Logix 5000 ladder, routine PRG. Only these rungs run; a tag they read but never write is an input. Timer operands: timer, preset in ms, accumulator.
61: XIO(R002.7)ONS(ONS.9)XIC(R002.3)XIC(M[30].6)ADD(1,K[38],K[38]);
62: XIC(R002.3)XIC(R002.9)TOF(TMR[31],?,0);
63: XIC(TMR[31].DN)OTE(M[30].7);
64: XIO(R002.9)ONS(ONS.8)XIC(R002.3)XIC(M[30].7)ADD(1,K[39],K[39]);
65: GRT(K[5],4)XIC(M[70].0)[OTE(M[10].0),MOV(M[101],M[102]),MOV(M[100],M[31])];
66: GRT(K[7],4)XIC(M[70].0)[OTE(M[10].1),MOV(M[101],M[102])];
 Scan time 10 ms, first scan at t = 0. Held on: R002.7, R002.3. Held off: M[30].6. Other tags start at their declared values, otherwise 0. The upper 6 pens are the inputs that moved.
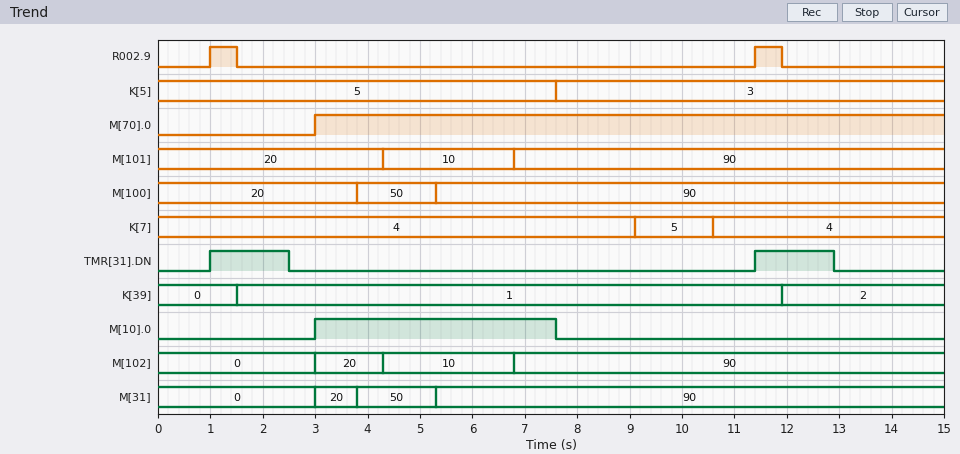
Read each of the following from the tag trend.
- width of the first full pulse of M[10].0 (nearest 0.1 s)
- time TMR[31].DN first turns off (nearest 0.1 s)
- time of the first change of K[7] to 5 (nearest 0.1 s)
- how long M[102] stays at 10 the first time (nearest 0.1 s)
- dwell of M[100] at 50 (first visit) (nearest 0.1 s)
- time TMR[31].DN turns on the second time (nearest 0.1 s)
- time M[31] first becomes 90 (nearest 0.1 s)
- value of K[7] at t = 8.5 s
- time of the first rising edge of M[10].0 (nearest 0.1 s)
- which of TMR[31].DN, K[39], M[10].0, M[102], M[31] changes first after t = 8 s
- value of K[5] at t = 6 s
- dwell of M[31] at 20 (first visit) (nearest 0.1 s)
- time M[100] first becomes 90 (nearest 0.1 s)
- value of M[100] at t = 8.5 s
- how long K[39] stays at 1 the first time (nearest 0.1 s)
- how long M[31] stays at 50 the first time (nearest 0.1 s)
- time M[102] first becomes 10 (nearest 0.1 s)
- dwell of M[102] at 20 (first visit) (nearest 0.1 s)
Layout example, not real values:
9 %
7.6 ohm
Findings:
4.6 s
2.5 s
9.1 s
2.5 s
1.5 s
11.4 s
5.3 s
4
3.0 s
TMR[31].DN
5
0.8 s
5.3 s
90
10.4 s
1.5 s
4.3 s
1.3 s
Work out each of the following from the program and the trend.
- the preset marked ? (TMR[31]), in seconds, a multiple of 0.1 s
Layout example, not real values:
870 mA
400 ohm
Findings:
1.0 s
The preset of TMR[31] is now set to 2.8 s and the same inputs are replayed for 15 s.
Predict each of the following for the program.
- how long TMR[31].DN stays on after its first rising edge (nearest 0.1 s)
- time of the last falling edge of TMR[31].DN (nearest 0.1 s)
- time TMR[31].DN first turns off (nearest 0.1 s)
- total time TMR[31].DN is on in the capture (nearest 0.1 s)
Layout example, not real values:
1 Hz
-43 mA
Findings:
3.3 s
14.7 s
4.3 s
6.6 s
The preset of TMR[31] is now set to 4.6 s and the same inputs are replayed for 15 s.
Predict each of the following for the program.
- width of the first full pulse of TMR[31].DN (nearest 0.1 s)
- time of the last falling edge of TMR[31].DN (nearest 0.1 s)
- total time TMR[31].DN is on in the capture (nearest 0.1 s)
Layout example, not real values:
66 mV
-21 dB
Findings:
5.1 s
6.1 s
8.7 s
